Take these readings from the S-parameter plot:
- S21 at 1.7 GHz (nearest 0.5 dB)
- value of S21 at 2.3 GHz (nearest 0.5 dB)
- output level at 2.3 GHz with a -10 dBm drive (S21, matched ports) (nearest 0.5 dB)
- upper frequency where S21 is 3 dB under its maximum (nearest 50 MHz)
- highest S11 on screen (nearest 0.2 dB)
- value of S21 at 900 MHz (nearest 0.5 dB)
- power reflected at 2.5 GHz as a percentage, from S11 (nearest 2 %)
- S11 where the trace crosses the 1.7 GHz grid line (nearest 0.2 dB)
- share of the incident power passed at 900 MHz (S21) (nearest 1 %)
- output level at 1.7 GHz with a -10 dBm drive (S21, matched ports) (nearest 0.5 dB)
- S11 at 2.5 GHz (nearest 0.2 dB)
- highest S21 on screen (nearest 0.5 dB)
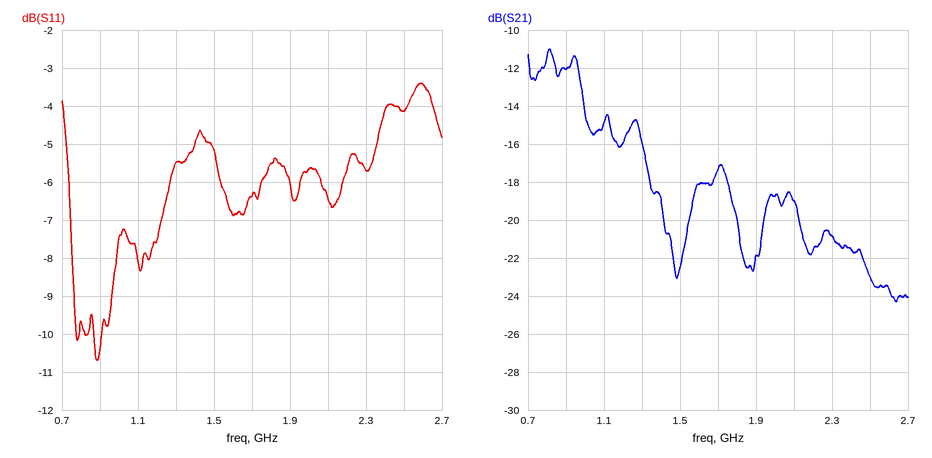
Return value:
-17.5 dB
-21.0 dB
-31.0 dBm
1.00 GHz
-3.4 dB
-12.0 dB
38 %
-6.4 dB
6 %
-27.5 dBm
-4.2 dB
-11.0 dB
